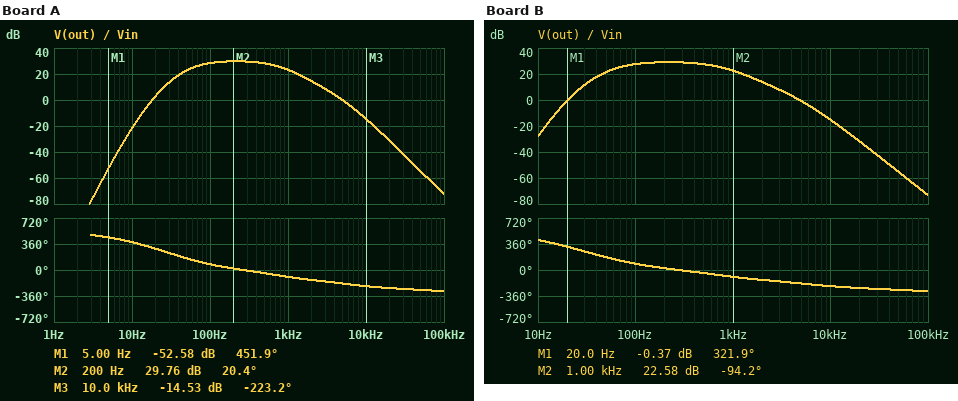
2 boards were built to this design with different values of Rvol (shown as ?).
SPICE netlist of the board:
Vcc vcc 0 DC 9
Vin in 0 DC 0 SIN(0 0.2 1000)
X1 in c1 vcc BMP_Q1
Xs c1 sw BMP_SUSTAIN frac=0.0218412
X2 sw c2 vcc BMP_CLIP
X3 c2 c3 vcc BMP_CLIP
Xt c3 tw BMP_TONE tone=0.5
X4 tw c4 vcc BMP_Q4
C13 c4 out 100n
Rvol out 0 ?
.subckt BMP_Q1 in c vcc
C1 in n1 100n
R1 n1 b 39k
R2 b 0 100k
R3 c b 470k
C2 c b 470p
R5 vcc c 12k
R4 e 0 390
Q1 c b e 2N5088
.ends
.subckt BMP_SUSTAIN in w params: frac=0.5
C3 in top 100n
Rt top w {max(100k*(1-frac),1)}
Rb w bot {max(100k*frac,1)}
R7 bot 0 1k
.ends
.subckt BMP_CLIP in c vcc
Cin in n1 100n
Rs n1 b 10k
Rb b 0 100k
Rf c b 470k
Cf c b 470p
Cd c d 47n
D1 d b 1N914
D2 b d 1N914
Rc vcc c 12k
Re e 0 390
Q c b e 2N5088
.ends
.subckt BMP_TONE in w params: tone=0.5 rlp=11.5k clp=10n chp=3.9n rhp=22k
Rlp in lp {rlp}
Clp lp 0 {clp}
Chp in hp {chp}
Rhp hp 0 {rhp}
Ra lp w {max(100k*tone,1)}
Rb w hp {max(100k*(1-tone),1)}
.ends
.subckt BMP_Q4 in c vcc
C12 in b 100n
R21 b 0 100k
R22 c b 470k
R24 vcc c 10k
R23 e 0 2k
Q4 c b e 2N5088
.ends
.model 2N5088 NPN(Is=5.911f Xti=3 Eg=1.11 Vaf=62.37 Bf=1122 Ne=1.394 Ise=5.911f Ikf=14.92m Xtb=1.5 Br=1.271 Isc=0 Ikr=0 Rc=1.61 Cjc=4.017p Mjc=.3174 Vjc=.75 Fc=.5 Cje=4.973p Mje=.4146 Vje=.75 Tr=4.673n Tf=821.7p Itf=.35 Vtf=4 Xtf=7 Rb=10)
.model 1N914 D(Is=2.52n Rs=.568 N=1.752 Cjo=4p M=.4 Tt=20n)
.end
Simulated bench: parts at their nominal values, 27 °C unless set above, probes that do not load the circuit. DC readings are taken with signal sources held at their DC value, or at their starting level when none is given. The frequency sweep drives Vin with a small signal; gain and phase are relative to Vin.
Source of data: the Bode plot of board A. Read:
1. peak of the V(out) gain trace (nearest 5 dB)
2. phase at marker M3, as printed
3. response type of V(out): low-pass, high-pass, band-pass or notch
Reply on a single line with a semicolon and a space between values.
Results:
30 dB; -223.2 deg; band-pass
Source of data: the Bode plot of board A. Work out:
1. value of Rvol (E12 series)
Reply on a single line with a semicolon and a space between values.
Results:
220 kΩ
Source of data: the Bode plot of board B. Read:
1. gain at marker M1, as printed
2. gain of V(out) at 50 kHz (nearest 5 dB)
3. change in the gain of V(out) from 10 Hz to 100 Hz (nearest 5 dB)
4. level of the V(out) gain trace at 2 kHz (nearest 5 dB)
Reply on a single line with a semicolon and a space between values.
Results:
-0.37 dB; -55 dB; 55 dB; 15 dB
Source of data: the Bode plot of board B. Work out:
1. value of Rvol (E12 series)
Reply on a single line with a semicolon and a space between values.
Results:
68 kΩ
